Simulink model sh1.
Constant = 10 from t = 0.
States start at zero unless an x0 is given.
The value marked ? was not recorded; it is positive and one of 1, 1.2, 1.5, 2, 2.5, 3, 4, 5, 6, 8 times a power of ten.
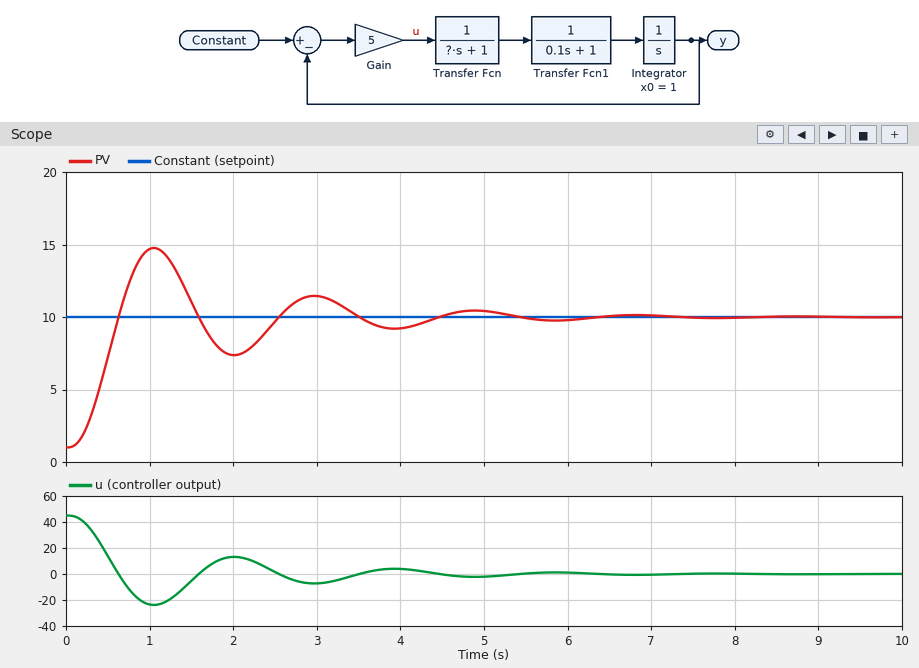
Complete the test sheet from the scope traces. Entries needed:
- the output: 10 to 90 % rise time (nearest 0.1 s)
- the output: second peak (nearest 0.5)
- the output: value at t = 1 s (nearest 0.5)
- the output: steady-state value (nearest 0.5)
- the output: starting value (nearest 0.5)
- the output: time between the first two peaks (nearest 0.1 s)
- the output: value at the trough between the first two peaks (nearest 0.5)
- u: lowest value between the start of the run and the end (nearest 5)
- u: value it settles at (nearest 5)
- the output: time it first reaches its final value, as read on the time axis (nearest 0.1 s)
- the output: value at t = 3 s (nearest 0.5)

0.4 s
11.5
14.5
10.0
1.0
1.9 s
7.5
-25
0
0.6 s
11.5
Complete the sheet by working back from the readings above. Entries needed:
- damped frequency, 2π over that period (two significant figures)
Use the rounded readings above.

3.3 rad/s
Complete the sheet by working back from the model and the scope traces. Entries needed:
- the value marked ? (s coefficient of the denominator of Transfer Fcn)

0.4
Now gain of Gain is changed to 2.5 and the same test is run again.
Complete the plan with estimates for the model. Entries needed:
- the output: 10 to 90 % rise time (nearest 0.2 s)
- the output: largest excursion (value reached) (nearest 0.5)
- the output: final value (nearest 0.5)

0.6 s
12.5
10.0
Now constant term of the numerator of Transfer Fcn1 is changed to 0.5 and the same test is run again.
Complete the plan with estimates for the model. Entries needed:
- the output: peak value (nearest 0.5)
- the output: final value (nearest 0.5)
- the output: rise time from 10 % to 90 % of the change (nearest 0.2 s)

12.5
10.0
0.6 s
